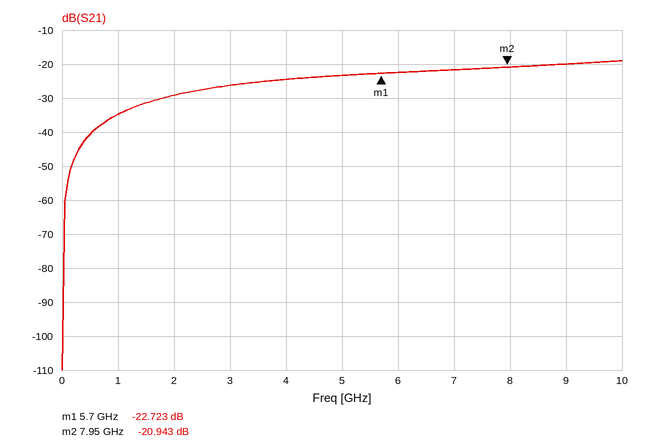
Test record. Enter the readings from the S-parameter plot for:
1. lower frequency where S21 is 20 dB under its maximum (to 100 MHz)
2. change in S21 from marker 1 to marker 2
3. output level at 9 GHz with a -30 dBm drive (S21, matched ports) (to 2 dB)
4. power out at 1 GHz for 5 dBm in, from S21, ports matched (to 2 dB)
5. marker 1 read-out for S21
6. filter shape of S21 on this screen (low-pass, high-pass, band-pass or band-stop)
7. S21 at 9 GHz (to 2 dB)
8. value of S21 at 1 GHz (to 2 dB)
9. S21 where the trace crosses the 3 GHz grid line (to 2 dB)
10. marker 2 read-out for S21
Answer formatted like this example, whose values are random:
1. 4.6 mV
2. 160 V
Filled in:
1. 600 MHz
2. 1.780 dB
3. -50 dBm
4. -30 dBm
5. -22.723 dB
6. high-pass
7. -20 dB
8. -34 dB
9. -26 dB
10. -20.943 dB
